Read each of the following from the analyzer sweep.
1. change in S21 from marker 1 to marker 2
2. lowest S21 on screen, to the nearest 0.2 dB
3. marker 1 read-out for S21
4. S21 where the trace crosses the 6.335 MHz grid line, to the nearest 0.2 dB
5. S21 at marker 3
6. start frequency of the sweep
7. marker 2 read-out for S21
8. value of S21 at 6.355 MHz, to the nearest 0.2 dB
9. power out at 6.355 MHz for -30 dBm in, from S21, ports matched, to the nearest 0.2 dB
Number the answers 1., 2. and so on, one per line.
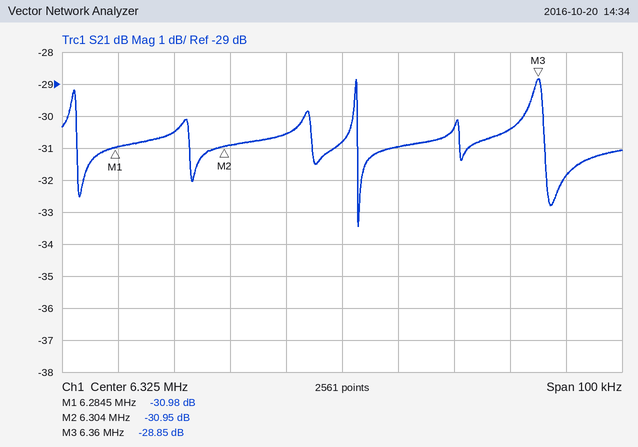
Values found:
1. 0.03 dB
2. -33.4 dB
3. -30.98 dB
4. -31.0 dB
5. -28.85 dB
6. 6.275 MHz
7. -30.95 dB
8. -30.4 dB
9. -60.4 dBm
